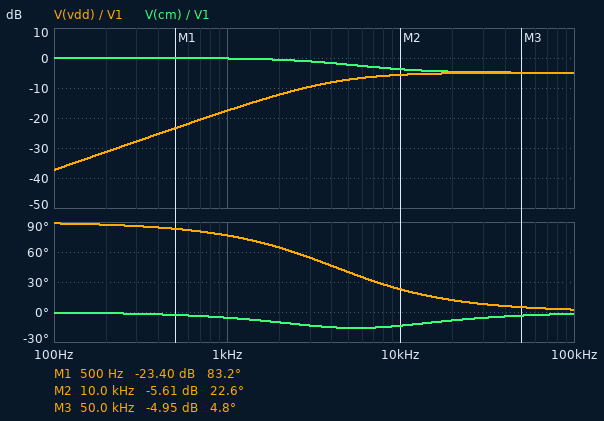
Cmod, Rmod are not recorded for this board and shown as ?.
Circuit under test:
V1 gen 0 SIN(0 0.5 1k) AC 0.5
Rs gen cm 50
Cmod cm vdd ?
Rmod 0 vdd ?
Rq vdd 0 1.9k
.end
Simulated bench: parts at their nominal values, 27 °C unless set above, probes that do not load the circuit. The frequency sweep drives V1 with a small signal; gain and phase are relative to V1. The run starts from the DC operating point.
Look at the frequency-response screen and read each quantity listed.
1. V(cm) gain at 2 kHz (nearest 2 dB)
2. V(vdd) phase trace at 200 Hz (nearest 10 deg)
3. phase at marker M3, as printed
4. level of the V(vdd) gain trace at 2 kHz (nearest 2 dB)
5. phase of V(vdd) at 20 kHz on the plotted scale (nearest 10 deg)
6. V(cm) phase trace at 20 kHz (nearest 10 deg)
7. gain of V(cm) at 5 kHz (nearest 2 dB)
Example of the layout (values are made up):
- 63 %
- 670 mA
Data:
- 0 dB
- 90 deg
- 4.8 deg
- -12 dB
- 10 deg
- -10 deg
- -2 dB
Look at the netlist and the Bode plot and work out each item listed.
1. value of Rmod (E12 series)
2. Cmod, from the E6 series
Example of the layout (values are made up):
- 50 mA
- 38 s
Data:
- 68 Ω
- 330 nF
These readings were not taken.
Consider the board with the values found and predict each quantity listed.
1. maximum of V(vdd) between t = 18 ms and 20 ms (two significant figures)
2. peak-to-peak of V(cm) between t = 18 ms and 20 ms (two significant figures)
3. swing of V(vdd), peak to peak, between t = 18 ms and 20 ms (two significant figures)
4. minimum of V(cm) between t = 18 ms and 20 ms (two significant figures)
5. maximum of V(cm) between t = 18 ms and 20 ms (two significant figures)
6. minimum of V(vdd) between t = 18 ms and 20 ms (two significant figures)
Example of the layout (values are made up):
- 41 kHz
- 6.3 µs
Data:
- 66 mV
- 980 mV
- 130 mV
- -490 mV
- 490 mV
- -66 mV
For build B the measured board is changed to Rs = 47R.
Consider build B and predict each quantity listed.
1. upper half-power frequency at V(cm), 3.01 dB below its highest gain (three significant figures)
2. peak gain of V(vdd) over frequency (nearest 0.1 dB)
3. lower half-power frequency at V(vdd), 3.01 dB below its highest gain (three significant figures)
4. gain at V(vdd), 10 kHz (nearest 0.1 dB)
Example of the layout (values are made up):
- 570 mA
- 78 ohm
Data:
- 7.56 kHz
- -4.7 dB
- 4.28 kHz
- -5.4 dB
